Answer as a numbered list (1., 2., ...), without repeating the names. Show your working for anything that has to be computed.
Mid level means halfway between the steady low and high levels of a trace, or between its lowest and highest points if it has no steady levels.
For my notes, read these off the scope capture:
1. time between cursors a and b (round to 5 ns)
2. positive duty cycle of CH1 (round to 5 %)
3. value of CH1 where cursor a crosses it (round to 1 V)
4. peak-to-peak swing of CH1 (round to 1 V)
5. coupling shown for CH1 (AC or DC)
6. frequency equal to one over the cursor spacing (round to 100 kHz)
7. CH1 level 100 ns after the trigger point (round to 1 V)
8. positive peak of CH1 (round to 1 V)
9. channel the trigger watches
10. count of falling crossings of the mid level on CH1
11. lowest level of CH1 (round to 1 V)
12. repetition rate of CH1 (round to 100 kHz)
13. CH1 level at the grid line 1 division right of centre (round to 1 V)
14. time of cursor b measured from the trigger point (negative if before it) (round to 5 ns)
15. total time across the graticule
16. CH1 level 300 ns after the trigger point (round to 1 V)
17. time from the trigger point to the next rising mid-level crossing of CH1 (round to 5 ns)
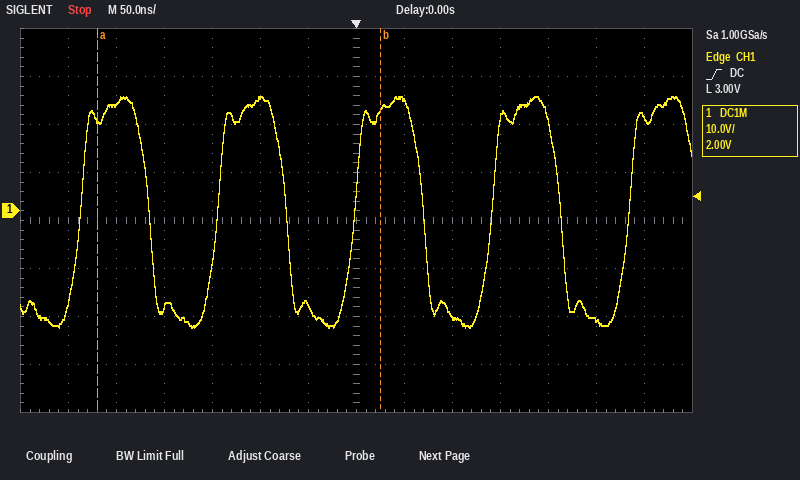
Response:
1. 295 ns
2. 50 %
3. 19 V
4. 24 V − (-24 V) = 48 V
5. DC
6. 1 / 295 ns ≈ 3.4 MHz
7. -22 V
8. 24 V
9. CH1
10. 4
11. -24 V
12. 7.0 MHz
13. 23 V
14. +25 ns
15. 700 ns
16. 20 V
17. 140 ns
